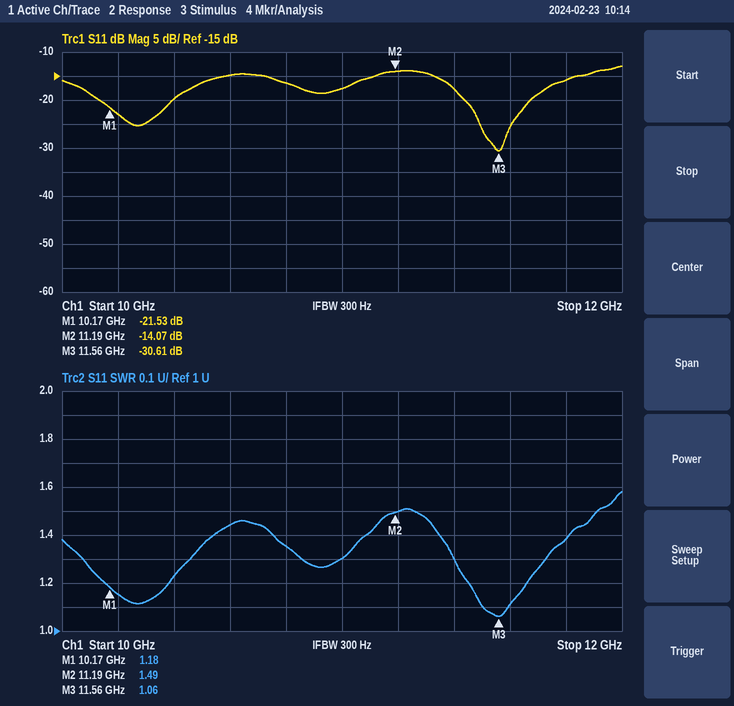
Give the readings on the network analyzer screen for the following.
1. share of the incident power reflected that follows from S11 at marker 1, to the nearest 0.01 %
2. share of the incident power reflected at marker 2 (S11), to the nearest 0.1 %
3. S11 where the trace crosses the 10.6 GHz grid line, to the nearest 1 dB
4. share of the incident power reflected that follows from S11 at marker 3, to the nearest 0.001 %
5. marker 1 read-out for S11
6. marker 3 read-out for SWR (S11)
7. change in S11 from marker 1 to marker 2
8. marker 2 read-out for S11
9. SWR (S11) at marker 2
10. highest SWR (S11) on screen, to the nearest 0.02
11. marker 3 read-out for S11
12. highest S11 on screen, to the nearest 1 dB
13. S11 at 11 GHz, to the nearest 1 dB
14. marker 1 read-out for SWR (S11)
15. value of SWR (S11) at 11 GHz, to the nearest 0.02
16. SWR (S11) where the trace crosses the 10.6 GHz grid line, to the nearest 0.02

0.70 %
3.9 %
-15 dB
0.087 %
-21.53 dB
1.06
7.46 dB
-14.07 dB
1.49
1.58
-30.61 dB
-13 dB
-18 dB
1.18
1.30
1.44
